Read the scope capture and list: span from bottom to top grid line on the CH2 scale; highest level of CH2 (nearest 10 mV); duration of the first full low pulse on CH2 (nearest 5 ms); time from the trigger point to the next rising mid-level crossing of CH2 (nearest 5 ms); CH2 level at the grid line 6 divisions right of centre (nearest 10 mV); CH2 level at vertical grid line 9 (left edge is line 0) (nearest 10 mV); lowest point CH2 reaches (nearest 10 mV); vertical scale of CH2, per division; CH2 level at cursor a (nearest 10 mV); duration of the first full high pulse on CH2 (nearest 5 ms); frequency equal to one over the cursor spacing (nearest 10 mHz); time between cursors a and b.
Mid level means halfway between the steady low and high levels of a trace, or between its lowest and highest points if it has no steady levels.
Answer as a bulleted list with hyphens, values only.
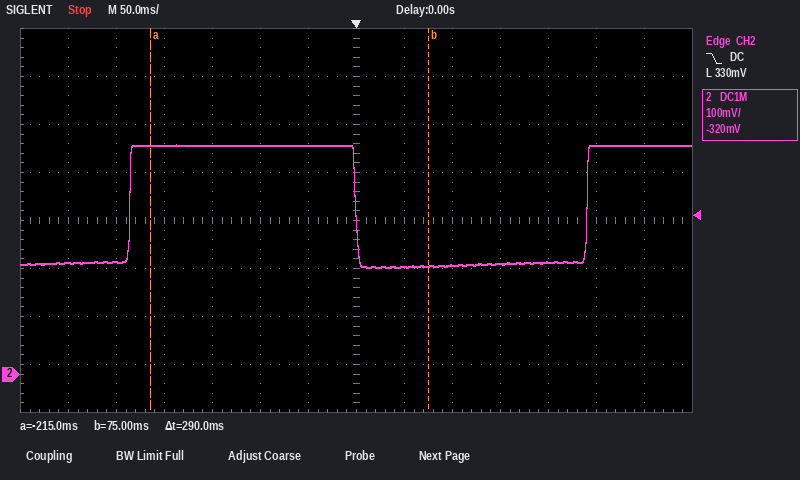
- 800 mV
- 480 mV
- 240 ms
- 240 ms
- 480 mV
- 230 mV
- 220 mV
- 100 mV
- 480 mV
- 235 ms
- 3.45 Hz
- 290 ms
